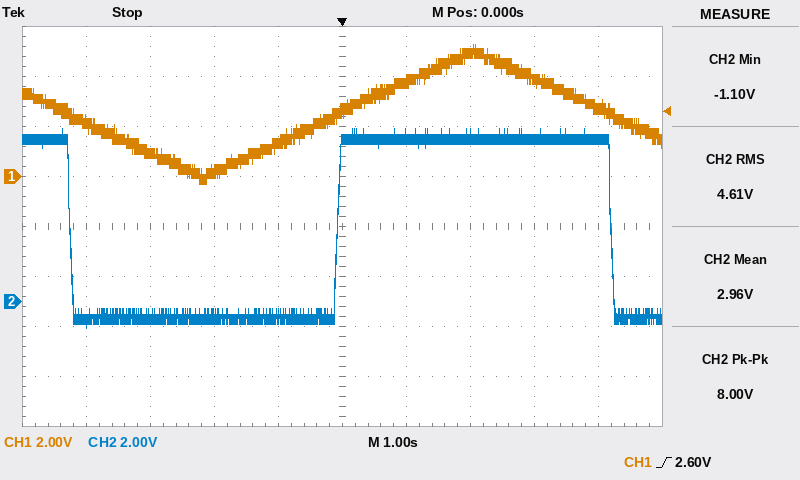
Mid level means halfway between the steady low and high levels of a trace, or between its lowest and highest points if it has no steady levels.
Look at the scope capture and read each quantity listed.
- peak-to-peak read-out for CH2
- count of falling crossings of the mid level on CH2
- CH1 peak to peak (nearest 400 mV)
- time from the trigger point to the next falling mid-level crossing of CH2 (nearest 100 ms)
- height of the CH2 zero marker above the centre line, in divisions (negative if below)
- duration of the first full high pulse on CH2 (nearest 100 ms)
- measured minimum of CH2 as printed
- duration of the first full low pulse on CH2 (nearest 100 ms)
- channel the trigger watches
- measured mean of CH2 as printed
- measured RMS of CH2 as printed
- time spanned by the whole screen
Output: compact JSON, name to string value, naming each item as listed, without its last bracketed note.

{"peak-to-peak read-out for CH2": "8.00 V", "count of falling crossings of the mid level on CH2": "2", "CH1 peak to peak": "5.6 V", "time from the trigger point to the next falling mid-level crossing of CH2": "4.2 s", "height of the CH2 zero marker above the centre line, in divisions": "-1.5 div", "duration of the first full high pulse on CH2": "4.3 s", "measured minimum of CH2 as printed": "-1.10 V", "duration of the first full low pulse on CH2": "4.2 s", "channel the trigger watches": "CH1", "measured mean of CH2 as printed": "2.96 V", "measured RMS of CH2 as printed": "4.61 V", "time spanned by the whole screen": "10 s"}
